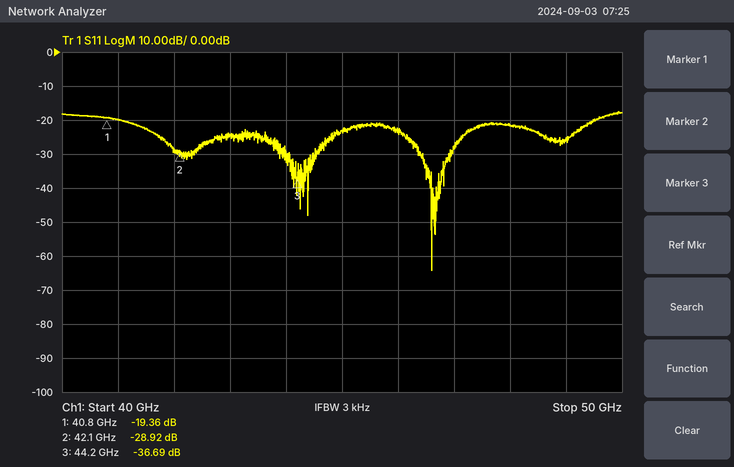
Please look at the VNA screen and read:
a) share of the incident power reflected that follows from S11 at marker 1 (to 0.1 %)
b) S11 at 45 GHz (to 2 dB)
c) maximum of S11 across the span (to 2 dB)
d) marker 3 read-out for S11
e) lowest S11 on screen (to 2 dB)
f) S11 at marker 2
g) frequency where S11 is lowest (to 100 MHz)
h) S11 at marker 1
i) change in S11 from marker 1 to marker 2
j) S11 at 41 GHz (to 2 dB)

1.2 %
-24 dB
-18 dB
-36.69 dB
-64 dB
-28.92 dB
46.6 GHz
-19.36 dB
-9.56 dB
-20 dB
